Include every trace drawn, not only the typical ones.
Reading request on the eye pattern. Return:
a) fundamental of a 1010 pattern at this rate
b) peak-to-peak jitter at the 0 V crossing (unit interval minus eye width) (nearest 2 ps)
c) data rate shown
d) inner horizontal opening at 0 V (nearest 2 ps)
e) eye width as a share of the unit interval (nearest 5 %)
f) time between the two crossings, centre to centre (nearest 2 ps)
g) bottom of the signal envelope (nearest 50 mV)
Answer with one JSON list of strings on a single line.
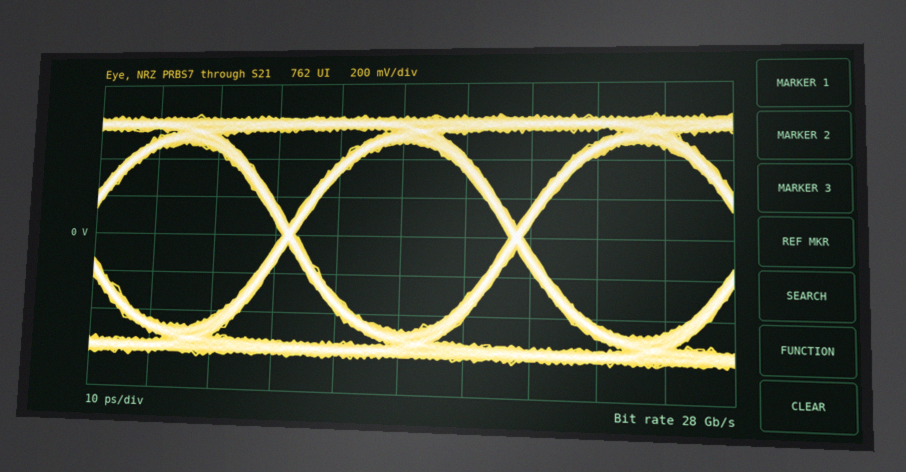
["14 GHz", "2 ps", "28 Gb/s", "34 ps", "95 %", "36 ps", "-650 mV"]
